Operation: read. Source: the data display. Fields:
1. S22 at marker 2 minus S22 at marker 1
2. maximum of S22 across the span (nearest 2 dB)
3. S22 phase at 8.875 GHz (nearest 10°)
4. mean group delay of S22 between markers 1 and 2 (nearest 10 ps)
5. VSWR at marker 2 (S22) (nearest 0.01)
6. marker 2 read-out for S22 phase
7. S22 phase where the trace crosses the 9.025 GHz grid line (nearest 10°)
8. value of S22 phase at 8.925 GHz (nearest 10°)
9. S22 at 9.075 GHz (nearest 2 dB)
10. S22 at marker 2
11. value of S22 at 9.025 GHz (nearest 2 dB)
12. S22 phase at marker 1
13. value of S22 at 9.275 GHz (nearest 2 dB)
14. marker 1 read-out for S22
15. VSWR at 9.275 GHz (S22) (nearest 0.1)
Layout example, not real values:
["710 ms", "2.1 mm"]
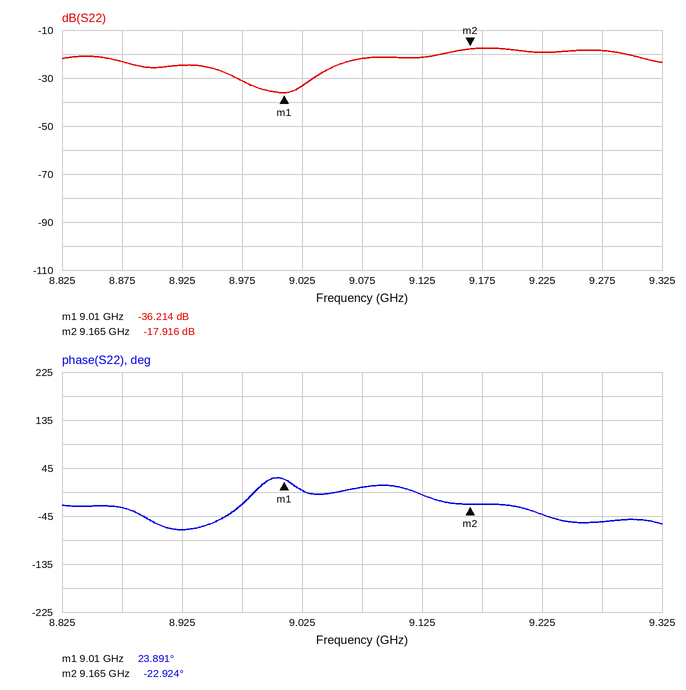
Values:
["18.298 dB", "-18 dB", "-30°", "840 ps", "1.29", "-22.924°", "0°", "-70°", "-22 dB", "-17.916 dB", "-34 dB", "23.891°", "-18 dB", "-36.214 dB", "1.3"]
